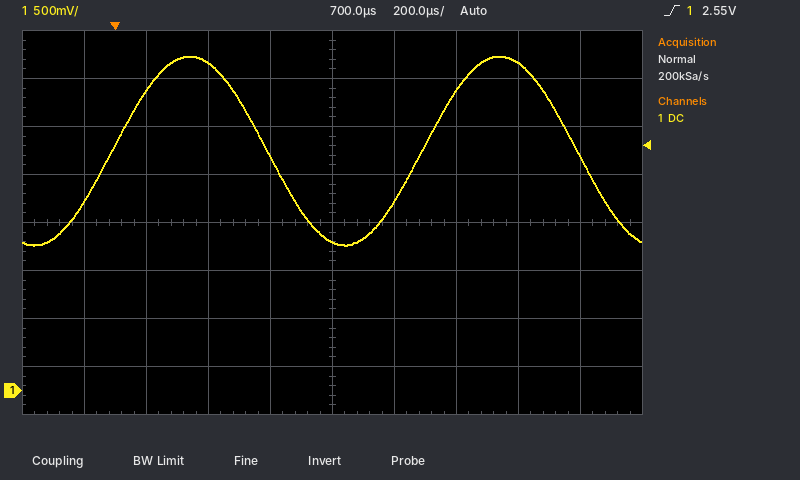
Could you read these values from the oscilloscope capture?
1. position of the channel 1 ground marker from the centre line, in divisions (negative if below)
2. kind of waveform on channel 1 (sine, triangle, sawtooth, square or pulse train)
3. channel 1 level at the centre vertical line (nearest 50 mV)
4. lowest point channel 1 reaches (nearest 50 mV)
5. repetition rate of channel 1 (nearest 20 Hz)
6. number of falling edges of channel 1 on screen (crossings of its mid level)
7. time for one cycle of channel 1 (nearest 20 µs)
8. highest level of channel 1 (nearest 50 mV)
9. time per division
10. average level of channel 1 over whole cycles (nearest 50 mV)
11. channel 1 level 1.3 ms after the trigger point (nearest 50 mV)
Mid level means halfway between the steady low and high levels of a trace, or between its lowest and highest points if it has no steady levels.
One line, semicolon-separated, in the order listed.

-3.5 div; sine; 1.55 V; 1.50 V; 1.00 kHz; 2; 1.00 ms; 3.50 V; 200 µs; 2.50 V; 3.40 V
